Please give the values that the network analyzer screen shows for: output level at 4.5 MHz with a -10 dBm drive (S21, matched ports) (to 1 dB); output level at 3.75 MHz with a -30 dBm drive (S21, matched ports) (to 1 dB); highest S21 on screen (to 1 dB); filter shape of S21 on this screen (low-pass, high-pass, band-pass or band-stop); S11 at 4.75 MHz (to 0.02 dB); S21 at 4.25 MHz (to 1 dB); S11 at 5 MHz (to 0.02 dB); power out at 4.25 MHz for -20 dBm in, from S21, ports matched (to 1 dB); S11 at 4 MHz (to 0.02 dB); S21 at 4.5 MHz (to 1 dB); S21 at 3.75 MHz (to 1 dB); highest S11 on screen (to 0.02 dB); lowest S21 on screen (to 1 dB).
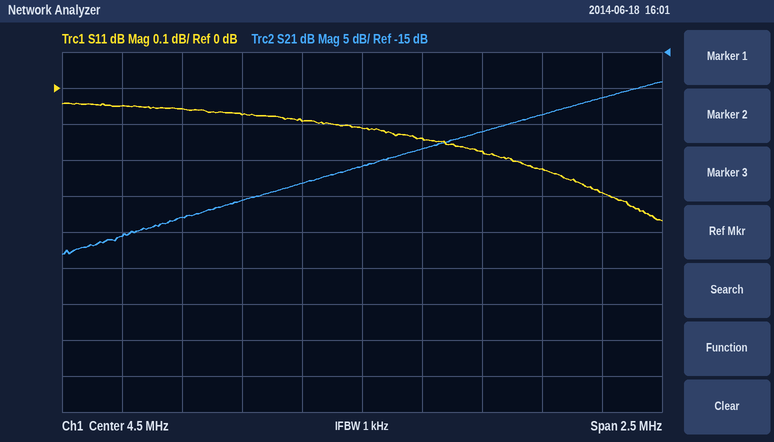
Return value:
-41 dBm
-68 dBm
-19 dB
high-pass
-0.14 dB
-33 dB
-0.18 dB
-53 dBm
-0.08 dB
-31 dB
-38 dB
-0.04 dB
-43 dB
